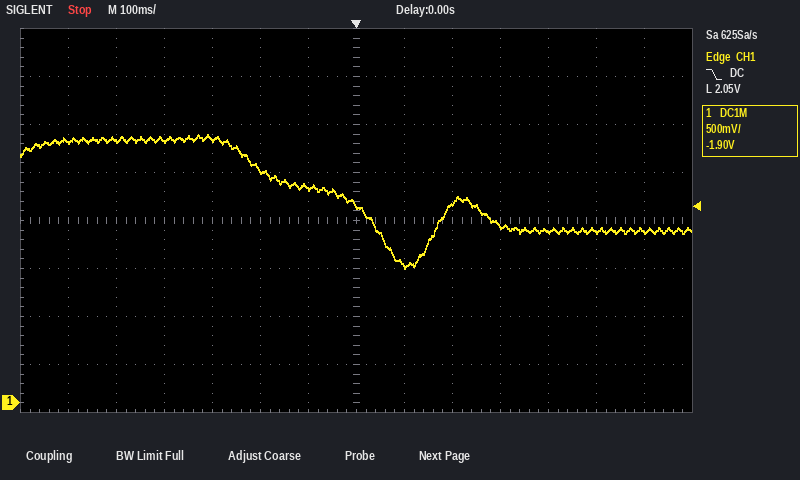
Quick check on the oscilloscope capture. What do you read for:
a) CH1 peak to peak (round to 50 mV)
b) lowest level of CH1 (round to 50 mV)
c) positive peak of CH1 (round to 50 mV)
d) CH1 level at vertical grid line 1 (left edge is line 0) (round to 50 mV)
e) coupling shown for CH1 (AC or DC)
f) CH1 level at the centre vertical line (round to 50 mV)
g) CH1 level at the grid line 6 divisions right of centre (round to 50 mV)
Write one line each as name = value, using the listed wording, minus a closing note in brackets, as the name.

CH1 peak to peak = 1.40 V
lowest level of CH1 = 1.40 V
positive peak of CH1 = 2.80 V
CH1 level at vertical grid line 1 (left edge is line 0) = 2.70 V
coupling shown for CH1 = DC
CH1 level at the centre vertical line = 2.05 V
CH1 level at the grid line 6 divisions right of centre = 1.80 V
